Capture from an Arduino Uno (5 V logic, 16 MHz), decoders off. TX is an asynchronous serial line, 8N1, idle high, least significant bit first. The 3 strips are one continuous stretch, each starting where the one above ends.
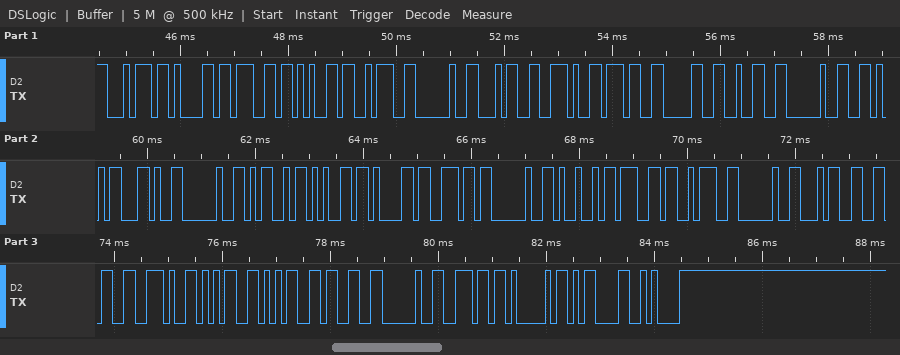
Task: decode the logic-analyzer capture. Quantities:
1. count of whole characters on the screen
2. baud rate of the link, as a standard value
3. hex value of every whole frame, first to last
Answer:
35
9600 baud
74 61 67 65 3A 20 34 2E 37 30 32 20 56 2C 20 4D 65 61 6E 20 49 67 3A 20 34 36 2E 35 35 33 20 6E 41 0D 0A
